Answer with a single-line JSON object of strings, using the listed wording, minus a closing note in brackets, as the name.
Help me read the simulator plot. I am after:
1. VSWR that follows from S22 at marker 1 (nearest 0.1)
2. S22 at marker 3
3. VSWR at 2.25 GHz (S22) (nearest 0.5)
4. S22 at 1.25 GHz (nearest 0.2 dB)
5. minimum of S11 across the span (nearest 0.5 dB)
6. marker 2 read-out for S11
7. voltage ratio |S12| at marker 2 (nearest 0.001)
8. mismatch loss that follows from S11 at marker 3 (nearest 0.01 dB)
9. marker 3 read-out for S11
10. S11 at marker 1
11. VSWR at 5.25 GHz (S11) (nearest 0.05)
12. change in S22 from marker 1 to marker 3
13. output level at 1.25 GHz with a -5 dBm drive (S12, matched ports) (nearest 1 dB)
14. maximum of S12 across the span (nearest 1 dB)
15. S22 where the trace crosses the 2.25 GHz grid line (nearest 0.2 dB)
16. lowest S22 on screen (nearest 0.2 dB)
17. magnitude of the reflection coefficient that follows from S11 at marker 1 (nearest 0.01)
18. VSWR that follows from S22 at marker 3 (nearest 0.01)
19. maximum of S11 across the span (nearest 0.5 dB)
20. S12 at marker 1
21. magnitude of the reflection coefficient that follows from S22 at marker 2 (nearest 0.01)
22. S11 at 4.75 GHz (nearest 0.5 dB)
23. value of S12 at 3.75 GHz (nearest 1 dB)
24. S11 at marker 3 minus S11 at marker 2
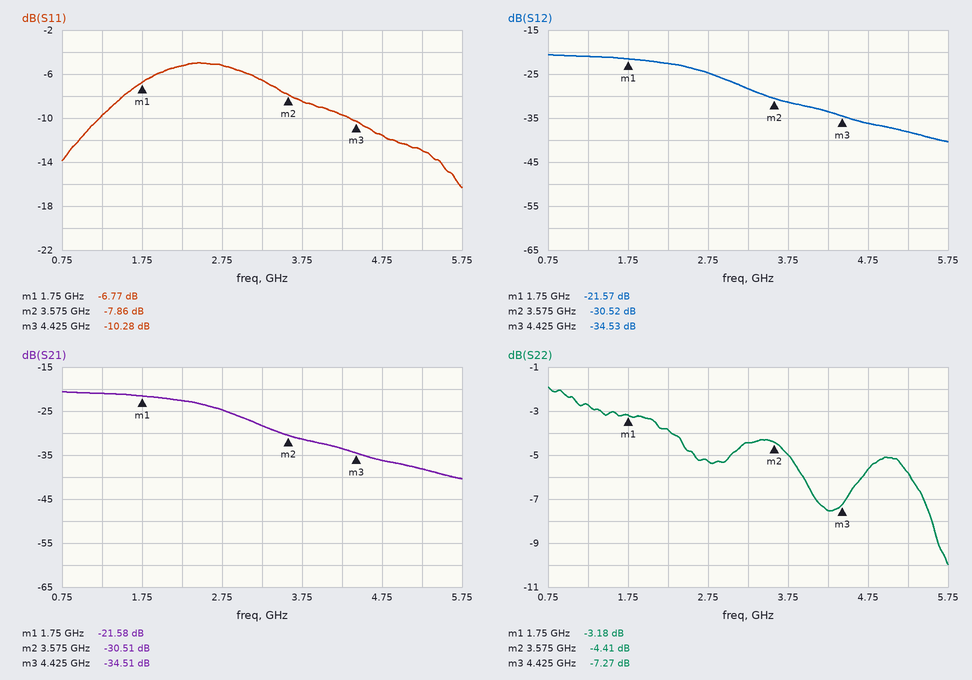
{"VSWR that follows from S22 at marker 1": "5.5", "S22 at marker 3": "-7.27 dB", "VSWR at 2.25 GHz (S22)": "4.5", "S22 at 1.25 GHz": "-2.8 dB", "minimum of S11 across the span": "-16.5 dB", "marker 2 read-out for S11": "-7.86 dB", "voltage ratio |S12| at marker 2": "0.030", "mismatch loss that follows from S11 at marker 3": "0.43 dB", "marker 3 read-out for S11": "-10.28 dB", "S11 at marker 1": "-6.77 dB", "VSWR at 5.25 GHz (S11)": "1.60", "change in S22 from marker 1 to marker 3": "-4.09 dB", "output level at 1.25 GHz with a -5 dBm drive (S12, matched ports)": "-26 dBm", "maximum of S12 across the span": "-21 dB", "S22 where the trace crosses the 2.25 GHz grid line": "-3.8 dB", "lowest S22 on screen": "-10.0 dB", "magnitude of the reflection coefficient that follows from S11 at marker 1": "0.46", "VSWR that follows from S22 at marker 3": "2.53", "maximum of S11 across the span": "-5.0 dB", "S12 at marker 1": "-21.57 dB", "magnitude of the reflection coefficient that follows from S22 at marker 2": "0.60", "S11 at 4.75 GHz": "-11.5 dB", "value of S12 at 3.75 GHz": "-31 dB", "S11 at marker 3 minus S11 at marker 2": "-2.42 dB"}
